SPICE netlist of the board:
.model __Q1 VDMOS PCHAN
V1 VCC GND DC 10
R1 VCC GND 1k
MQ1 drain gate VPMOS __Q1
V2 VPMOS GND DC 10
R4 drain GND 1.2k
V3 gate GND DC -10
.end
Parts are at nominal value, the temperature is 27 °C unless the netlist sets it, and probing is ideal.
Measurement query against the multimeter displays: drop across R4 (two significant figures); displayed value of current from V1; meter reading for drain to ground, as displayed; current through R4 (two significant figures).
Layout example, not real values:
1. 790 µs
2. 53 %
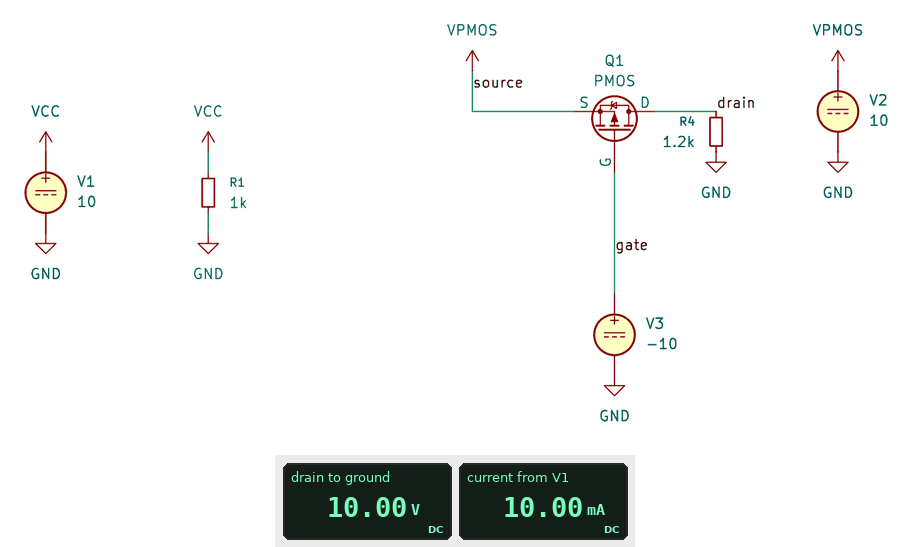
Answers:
1. 10 V
2. 10.00 mA
3. 10.00 V
4. 8.3 mA
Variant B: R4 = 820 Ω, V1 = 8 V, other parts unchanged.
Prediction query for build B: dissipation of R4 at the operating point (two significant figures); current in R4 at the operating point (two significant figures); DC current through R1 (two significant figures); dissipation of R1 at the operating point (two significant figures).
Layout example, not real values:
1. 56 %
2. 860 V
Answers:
1. 120 mW
2. 12 mA
3. 8.0 mA
4. 64 mW
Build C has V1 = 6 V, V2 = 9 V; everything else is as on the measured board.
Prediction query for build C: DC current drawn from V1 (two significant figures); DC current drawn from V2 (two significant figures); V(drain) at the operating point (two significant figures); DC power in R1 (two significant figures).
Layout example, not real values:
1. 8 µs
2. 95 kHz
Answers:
1. 6.0 mA
2. 7.5 mA
3. 9.0 V
4. 36 mW
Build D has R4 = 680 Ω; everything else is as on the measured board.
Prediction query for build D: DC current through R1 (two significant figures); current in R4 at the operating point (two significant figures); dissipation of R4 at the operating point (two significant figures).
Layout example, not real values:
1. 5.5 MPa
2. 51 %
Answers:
1. 10 mA
2. 15 mA
3. 150 mW
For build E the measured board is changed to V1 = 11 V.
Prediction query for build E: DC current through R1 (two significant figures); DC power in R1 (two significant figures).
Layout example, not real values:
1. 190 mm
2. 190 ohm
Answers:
1. 11 mA
2. 120 mW
